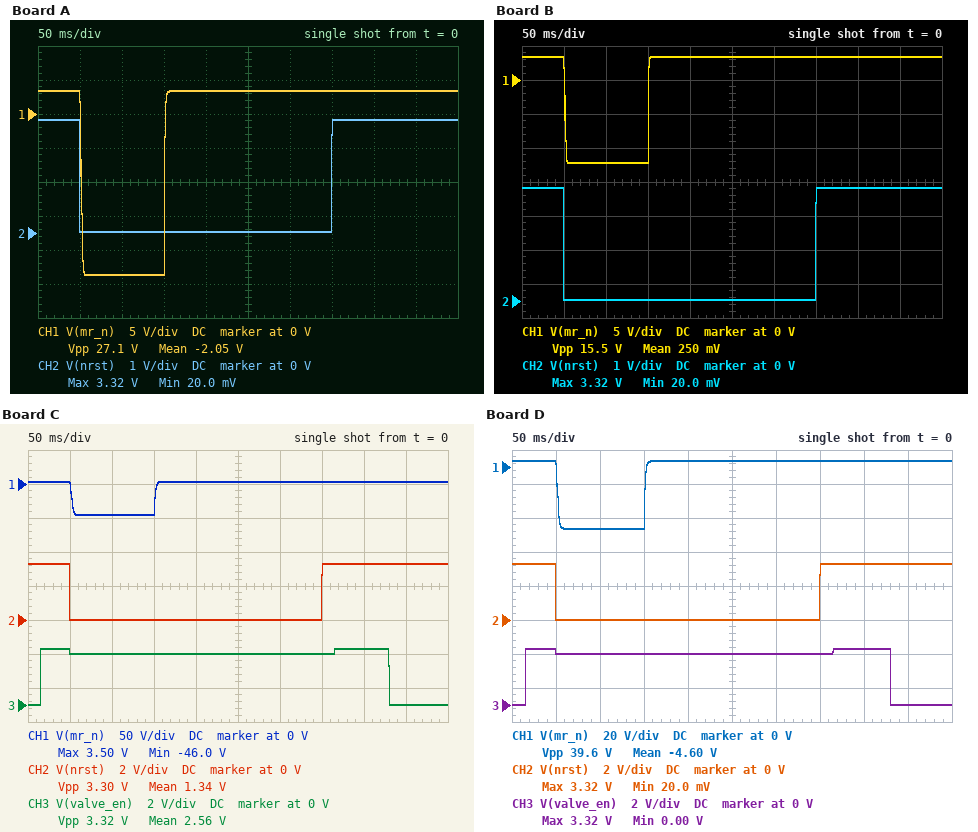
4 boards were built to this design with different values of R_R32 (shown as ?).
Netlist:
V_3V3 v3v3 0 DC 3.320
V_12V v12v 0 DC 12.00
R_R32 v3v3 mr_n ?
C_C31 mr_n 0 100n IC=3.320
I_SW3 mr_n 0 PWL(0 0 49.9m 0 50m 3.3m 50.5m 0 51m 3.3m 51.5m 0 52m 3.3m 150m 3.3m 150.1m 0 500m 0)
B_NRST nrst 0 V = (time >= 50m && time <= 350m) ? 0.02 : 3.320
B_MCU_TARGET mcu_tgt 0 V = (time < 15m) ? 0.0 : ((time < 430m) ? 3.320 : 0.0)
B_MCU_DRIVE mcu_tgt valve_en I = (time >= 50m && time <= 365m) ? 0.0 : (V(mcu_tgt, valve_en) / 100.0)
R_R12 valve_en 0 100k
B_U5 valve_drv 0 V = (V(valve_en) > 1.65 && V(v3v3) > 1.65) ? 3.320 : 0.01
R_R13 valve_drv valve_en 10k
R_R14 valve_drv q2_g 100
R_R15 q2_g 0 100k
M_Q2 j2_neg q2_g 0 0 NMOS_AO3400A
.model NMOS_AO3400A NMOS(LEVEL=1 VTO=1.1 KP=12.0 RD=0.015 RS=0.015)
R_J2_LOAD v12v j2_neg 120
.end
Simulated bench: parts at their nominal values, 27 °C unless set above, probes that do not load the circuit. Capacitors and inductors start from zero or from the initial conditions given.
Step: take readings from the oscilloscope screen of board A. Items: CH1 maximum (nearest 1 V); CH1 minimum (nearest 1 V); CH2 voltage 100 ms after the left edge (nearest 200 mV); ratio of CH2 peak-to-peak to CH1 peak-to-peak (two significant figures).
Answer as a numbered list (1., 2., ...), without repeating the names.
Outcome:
1. 3 V
2. -24 V
3. 0 V
4. 0.12
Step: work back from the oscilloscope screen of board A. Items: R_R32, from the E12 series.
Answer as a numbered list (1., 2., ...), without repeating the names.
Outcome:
1. 8.2 kΩ
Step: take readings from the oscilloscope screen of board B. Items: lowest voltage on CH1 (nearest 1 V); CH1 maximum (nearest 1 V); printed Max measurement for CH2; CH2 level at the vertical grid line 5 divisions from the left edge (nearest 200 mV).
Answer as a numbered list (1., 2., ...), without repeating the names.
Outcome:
1. -12 V
2. 3 V
3. 3.32 V
4. 0 V
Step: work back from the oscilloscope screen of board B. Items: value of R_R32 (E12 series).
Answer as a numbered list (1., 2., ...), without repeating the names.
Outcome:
1. 4.7 kΩ
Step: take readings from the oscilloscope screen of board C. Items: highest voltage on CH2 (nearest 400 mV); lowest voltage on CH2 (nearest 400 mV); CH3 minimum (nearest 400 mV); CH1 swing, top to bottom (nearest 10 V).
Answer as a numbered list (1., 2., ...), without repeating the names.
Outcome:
1. 3.2 V
2. 0 V
3. 0 V
4. 50 V
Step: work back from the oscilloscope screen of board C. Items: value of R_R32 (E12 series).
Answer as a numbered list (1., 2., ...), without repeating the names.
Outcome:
1. 15 kΩ
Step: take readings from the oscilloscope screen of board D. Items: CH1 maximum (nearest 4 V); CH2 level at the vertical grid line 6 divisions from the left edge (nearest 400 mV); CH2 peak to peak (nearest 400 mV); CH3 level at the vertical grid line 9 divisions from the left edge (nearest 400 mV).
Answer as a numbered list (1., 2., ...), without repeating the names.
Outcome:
1. 4 V
2. 0 V
3. 3.2 V
4. 0 V
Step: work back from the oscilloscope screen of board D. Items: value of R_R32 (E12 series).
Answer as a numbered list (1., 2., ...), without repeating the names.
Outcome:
1. 12 kΩ
